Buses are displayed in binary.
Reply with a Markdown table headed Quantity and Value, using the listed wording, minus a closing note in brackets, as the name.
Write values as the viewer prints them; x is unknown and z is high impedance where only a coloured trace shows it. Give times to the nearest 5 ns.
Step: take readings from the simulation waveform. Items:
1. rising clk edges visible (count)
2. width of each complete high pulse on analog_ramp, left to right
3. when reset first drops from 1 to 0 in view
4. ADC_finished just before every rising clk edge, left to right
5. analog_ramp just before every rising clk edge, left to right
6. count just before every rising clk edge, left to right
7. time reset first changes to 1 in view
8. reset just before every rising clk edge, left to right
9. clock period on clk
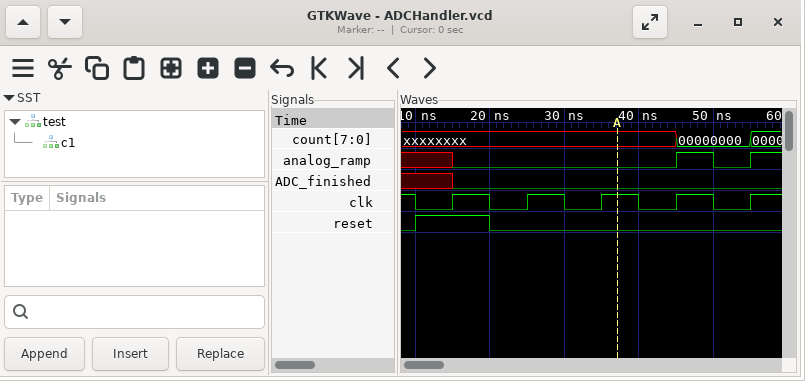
| Quantity | Value |
|---|---|
| rising clk edges visible | 5 |
| width of each complete high pulse on analog_ramp, left to right | 5 ns |
| when reset first drops from 1 to 0 in view | 20 ns |
| ADC_finished just before every rising clk edge, left to right | x 0 0 0 0 |
| analog_ramp just before every rising clk edge, left to right | x 0 0 0 0 |
| count just before every rising clk edge, left to right | xxxxxxxx, xxxxxxxx, xxxxxxxx, xxxxxxxx, 00000000 |
| time reset first changes to 1 in view | 10 ns |
| reset just before every rising clk edge, left to right | 1 0 0 0 0 |
| clock period on clk | 10 ns |
